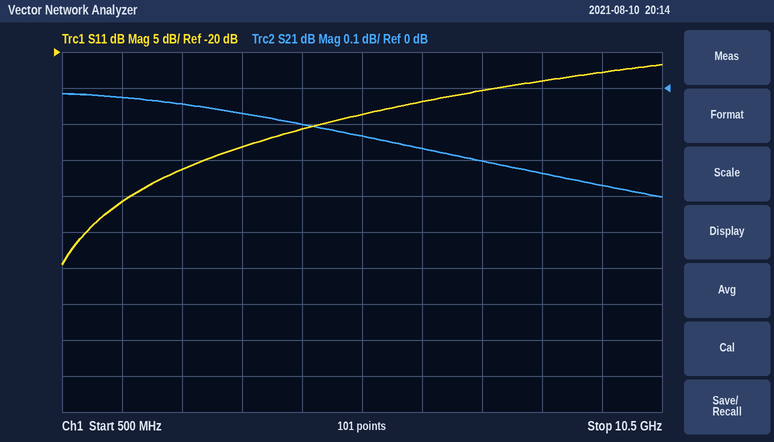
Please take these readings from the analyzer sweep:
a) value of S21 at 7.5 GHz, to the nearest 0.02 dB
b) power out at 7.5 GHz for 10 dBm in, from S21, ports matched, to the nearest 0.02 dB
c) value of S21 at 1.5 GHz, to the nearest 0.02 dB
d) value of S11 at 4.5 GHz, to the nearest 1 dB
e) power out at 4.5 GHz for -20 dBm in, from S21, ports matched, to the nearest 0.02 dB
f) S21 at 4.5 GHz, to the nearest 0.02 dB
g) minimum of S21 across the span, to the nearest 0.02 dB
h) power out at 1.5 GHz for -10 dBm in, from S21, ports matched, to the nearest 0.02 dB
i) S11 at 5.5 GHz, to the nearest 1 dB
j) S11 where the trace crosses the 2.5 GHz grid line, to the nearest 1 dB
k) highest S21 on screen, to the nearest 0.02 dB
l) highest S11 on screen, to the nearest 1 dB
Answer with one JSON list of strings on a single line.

["-0.20 dB", "9.80 dBm", "-0.02 dB", "-31 dB", "-20.10 dBm", "-0.10 dB", "-0.30 dB", "-10.02 dBm", "-29 dB", "-36 dB", "-0.02 dB", "-22 dB"]
